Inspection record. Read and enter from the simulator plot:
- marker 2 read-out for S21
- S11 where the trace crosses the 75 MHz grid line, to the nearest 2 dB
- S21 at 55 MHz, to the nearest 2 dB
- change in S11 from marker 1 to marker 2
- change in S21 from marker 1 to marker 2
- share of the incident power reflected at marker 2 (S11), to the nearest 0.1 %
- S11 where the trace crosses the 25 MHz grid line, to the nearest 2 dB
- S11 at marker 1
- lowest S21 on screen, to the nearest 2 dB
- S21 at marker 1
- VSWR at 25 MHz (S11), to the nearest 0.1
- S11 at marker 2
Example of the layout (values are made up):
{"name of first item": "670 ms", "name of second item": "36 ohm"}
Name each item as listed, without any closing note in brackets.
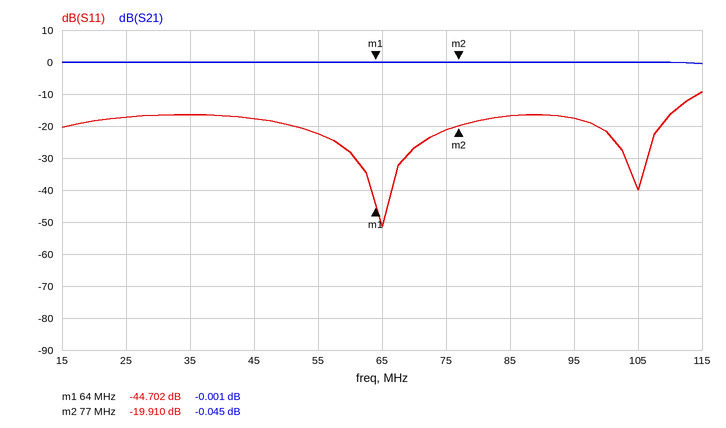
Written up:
{"marker 2 read-out for S21": "-0.045 dB", "S11 where the trace crosses the 75 MHz grid line, to the nearest 2 dB": "-22 dB", "S21 at 55 MHz, to the nearest 2 dB": "0 dB", "change in S11 from marker 1 to marker 2": "24.792 dB", "change in S21 from marker 1 to marker 2": "-0.044 dB", "share of the incident power reflected at marker 2 (S11), to the nearest 0.1 %": "1.0 %", "S11 where the trace crosses the 25 MHz grid line, to the nearest 2 dB": "-18 dB", "S11 at marker 1": "-44.702 dB", "lowest S21 on screen, to the nearest 2 dB": "0 dB", "S21 at marker 1": "-0.001 dB", "VSWR at 25 MHz (S11), to the nearest 0.1": "1.3", "S11 at marker 2": "-19.910 dB"}
